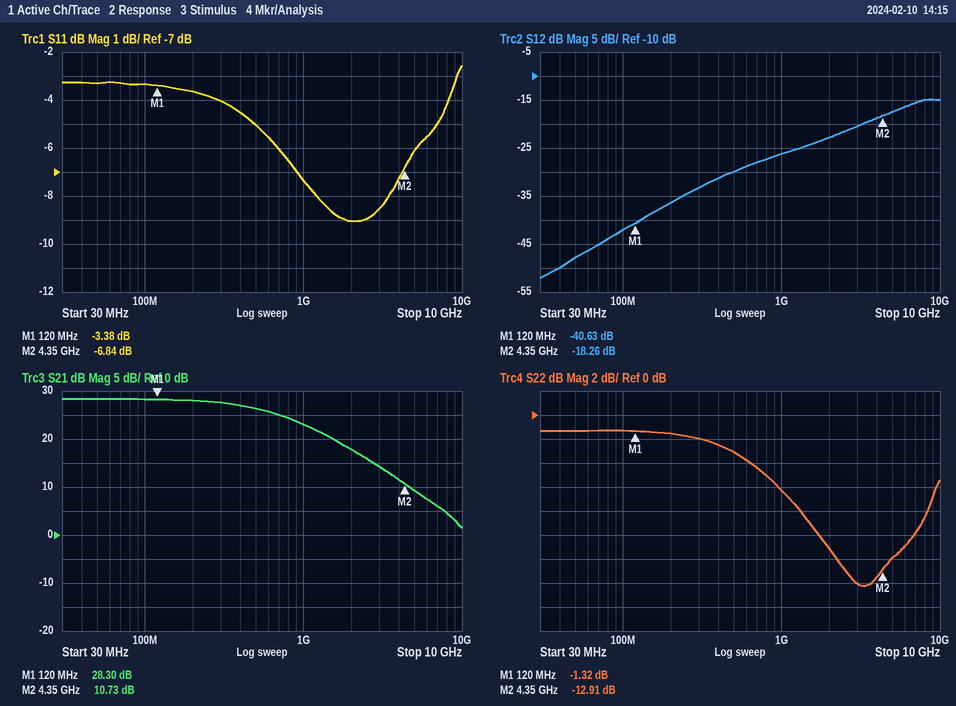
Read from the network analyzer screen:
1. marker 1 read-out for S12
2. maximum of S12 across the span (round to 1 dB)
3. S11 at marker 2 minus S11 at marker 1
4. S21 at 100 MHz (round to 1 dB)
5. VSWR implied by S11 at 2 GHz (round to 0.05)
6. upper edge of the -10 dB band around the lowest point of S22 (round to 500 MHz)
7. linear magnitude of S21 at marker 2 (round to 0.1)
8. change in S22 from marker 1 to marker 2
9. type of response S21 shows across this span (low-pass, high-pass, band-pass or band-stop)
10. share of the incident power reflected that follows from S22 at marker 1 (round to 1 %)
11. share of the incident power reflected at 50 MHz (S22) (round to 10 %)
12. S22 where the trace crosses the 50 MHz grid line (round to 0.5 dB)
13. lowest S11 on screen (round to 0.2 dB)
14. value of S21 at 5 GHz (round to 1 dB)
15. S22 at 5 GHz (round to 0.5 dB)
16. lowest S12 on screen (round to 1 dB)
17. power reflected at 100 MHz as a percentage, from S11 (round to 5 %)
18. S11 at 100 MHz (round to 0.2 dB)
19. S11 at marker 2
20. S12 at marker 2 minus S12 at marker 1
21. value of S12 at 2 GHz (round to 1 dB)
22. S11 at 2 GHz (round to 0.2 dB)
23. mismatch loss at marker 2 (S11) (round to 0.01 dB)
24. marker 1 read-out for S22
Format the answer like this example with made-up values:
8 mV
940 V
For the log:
-40.63 dB
-15 dB
-3.46 dB
28 dB
2.10
7.0 GHz
3.4
-11.59 dB
low-pass
74 %
70 %
-1.5 dB
-9.0 dB
9 dB
-12.0 dB
-52 dB
45 %
-3.4 dB
-6.84 dB
22.37 dB
-23 dB
-9.0 dB
1.01 dB
-1.32 dB
